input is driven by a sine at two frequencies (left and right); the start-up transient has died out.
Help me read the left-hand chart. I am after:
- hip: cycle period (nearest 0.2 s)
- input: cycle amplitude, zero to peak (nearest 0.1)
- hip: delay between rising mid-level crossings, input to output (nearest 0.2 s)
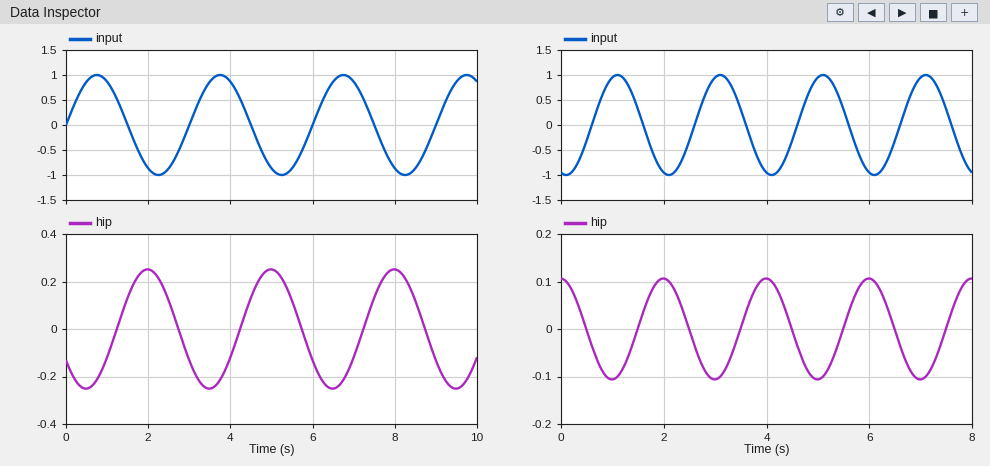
3.0 s
1.0
1.2 s
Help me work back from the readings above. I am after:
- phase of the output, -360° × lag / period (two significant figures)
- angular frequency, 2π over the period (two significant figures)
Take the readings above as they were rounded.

-140°
2.1 rad/s
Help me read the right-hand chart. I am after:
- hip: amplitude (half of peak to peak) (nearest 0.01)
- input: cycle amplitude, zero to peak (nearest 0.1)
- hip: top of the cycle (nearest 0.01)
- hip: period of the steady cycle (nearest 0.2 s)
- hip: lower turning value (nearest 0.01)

0.11
1.0
0.11
2.0 s
-0.11
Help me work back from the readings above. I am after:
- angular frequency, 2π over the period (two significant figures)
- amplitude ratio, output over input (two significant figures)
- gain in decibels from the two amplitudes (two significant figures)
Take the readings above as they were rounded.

3.1 rad/s
0.11
-19 dB
